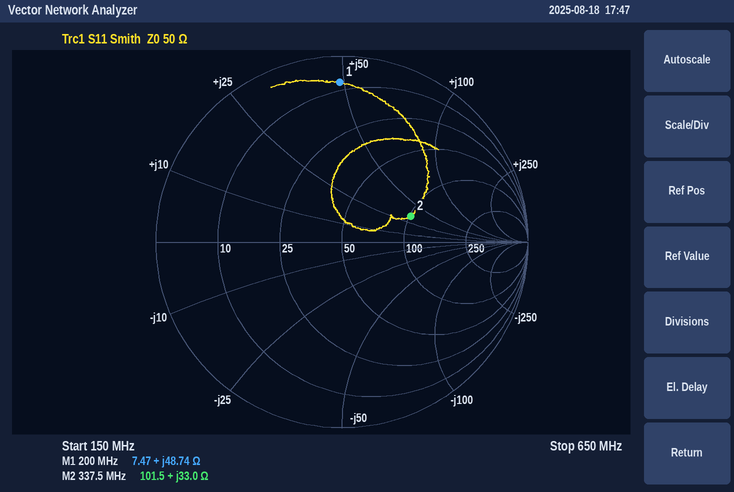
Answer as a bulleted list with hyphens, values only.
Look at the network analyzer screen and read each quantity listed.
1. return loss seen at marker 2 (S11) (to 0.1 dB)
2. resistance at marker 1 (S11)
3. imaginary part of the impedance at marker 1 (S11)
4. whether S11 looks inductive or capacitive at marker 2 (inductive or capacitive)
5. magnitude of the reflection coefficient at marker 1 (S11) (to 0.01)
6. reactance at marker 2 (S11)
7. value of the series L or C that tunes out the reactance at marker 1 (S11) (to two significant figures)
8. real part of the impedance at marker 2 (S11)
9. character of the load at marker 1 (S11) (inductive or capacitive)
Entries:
- 8.1 dB
- 7.47 Ω
- +48.74 Ω
- inductive
- 0.86
- +33.0 Ω
- 16 pF
- 101.5 Ω
- inductive
